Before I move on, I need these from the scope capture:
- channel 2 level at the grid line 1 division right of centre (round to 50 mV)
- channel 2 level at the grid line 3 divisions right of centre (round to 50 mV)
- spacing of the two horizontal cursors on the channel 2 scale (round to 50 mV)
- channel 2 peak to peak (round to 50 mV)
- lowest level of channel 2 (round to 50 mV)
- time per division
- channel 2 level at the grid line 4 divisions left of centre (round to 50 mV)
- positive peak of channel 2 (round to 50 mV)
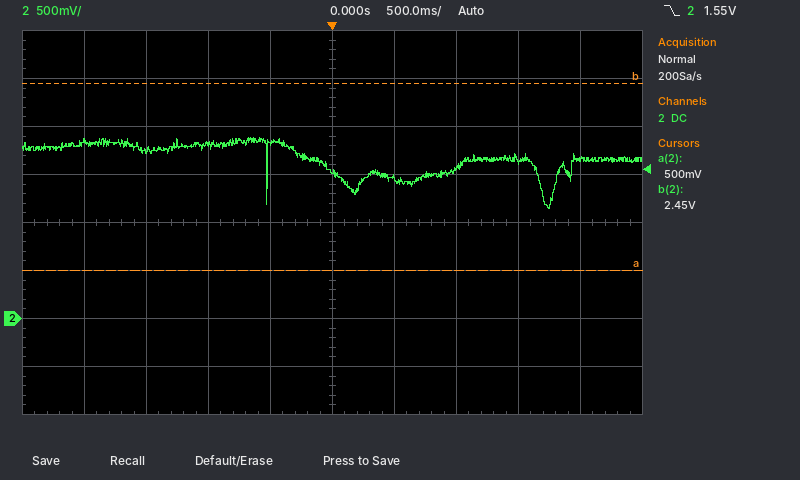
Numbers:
1.45 V
1.65 V
1.95 V
750 mV
1.15 V
500 ms
1.85 V
1.90 V
